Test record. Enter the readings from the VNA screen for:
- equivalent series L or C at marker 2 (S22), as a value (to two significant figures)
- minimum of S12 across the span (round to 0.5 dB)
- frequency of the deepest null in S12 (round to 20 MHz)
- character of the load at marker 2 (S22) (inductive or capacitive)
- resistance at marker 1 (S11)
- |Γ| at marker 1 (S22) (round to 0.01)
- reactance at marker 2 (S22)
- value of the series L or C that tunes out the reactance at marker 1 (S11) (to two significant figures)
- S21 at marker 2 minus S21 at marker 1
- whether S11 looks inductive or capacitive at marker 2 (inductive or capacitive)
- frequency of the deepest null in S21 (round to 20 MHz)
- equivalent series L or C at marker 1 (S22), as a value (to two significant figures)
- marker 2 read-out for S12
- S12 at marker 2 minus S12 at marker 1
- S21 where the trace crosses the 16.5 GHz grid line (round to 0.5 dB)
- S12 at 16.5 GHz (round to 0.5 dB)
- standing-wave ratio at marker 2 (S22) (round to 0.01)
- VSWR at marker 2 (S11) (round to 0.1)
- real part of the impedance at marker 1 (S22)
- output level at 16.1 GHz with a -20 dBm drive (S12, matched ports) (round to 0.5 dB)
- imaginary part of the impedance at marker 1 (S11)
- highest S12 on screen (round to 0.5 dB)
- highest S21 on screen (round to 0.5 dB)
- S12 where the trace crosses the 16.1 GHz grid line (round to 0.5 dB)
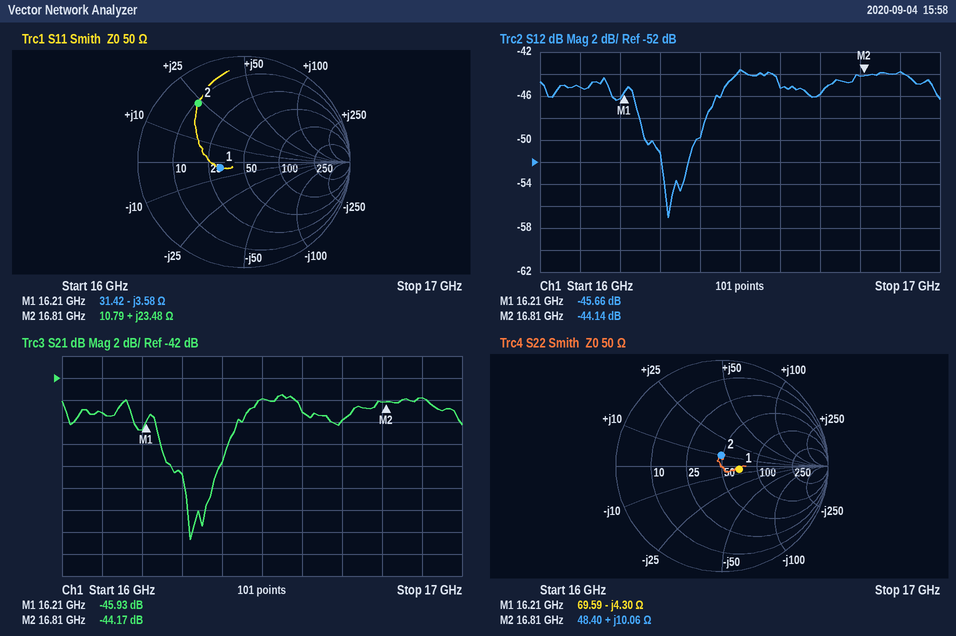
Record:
95 pH
-57.0 dB
16.32 GHz
inductive
31.42 Ω
0.17
+10.06 Ω
35 pH
1.76 dB
inductive
16.32 GHz
2.3 pF
-44.14 dB
1.52 dB
-44.0 dB
-43.5 dB
1.23
5.7
69.59 Ω
-65.0 dBm
-3.58 Ω
-43.5 dB
-43.5 dB
-45.0 dB
